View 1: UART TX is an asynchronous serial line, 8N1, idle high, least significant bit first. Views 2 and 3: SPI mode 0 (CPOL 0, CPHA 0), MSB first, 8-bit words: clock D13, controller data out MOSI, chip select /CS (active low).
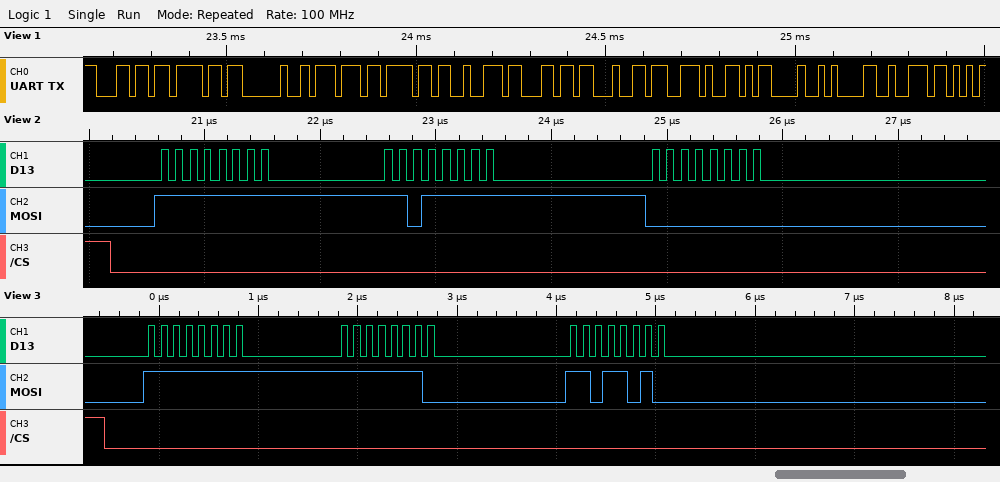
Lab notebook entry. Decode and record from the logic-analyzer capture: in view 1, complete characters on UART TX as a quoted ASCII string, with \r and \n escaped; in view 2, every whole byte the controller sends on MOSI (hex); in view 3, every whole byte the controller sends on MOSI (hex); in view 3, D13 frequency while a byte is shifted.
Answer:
"lo world.\r\nr"
FF DF 00
0xFF 0xFE 0xDA
8 MHz
